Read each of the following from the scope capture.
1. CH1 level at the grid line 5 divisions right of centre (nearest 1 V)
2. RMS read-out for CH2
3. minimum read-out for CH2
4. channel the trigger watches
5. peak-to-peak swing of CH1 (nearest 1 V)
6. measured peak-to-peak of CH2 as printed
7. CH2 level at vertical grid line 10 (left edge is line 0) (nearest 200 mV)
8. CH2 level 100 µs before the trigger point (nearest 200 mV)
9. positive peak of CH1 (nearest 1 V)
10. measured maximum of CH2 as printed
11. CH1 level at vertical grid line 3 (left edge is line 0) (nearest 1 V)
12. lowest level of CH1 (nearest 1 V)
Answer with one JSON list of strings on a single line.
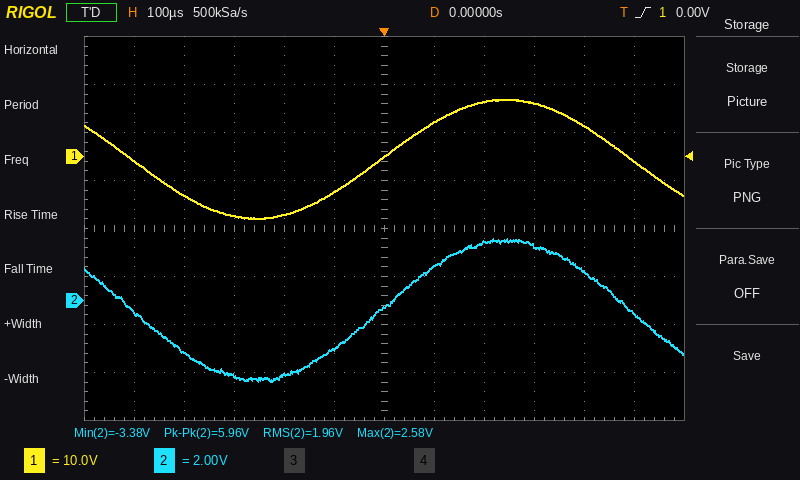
["-1 V", "1.96 V", "-3.38 V", "CH1", "25 V", "5.96 V", "1.2 V", "-2.0 V", "12 V", "2.58 V", "-12 V", "-13 V"]
